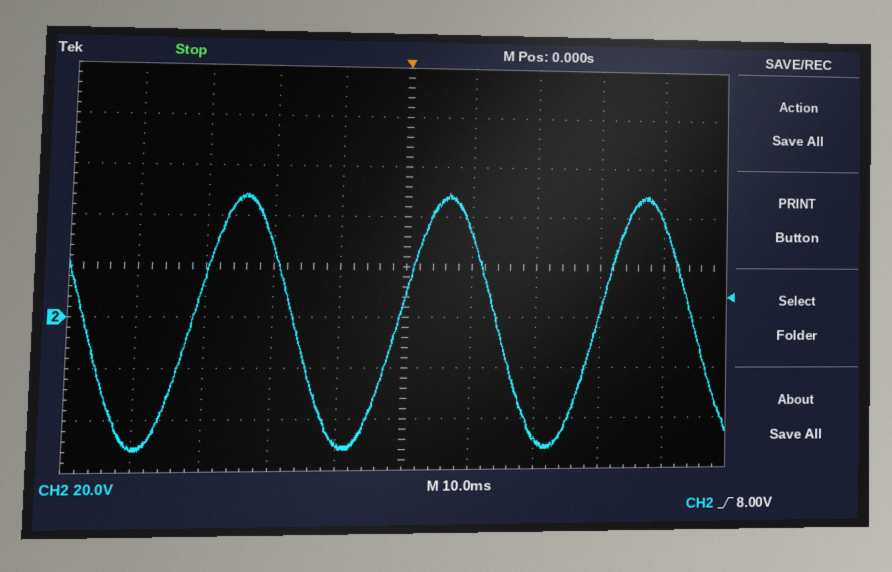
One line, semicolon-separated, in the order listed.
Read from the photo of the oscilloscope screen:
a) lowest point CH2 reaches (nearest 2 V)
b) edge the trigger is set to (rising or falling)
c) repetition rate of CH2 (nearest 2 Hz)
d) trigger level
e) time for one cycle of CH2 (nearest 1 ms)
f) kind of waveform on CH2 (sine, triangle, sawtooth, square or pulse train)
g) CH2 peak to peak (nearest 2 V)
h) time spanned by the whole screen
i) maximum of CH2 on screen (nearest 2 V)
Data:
-52 V; rising; 32 Hz; 8.00 V; 31 ms; sine; 102 V; 100 ms; 50 V
